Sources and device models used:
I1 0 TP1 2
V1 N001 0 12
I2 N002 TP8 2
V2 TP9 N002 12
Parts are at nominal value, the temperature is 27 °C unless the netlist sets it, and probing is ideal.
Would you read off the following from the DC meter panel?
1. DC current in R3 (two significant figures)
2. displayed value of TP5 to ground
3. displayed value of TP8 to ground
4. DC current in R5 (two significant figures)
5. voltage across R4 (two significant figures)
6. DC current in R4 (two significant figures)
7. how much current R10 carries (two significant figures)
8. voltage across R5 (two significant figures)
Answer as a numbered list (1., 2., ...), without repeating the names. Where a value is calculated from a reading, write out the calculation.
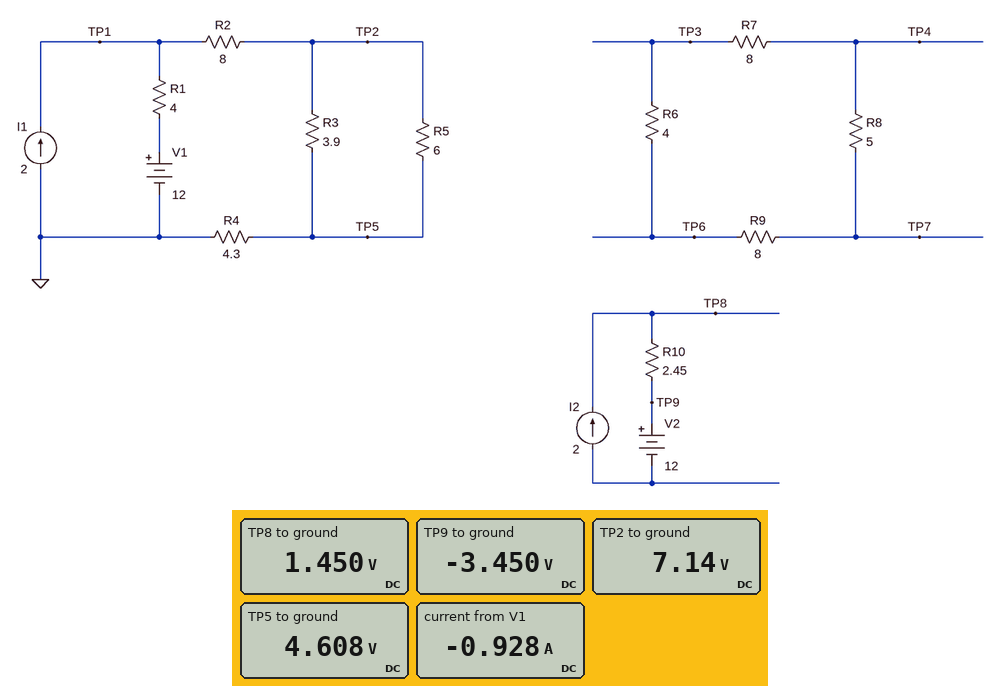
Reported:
1. (7.14 V - 4.608 V) / 3.9 Ω = 650 mA
2. 4.608 V
3. 1.450 V
4. (7.14 V - 4.608 V) / 6 Ω = 420 mA
5. 4.608 V = 4.6 V
6. (4.608 V) / 4.3 Ω = 1.1 A
7. (1.45 V - (-3.45 V)) / 2.45 Ω = 2.0 A
8. 7.14 V - 4.608 V = 2.5 V
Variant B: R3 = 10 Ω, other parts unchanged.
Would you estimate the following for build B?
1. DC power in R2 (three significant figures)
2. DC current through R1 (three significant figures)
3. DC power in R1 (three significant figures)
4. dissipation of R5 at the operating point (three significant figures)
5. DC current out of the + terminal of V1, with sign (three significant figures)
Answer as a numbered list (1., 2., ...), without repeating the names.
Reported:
1. 7.96 W
2. 1.00 A
3. 4.02 W
4. 2.33 W
5. -1.00 A
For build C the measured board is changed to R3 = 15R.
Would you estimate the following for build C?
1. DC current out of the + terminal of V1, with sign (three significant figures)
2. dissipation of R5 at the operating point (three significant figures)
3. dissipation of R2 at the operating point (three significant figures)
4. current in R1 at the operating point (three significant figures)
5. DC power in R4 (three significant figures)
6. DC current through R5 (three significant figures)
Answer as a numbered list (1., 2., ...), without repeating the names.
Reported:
1. -1.03 A
2. 2.89 W
3. 7.55 W
4. 1.03 A
5. 4.06 W
6. 694 mA
